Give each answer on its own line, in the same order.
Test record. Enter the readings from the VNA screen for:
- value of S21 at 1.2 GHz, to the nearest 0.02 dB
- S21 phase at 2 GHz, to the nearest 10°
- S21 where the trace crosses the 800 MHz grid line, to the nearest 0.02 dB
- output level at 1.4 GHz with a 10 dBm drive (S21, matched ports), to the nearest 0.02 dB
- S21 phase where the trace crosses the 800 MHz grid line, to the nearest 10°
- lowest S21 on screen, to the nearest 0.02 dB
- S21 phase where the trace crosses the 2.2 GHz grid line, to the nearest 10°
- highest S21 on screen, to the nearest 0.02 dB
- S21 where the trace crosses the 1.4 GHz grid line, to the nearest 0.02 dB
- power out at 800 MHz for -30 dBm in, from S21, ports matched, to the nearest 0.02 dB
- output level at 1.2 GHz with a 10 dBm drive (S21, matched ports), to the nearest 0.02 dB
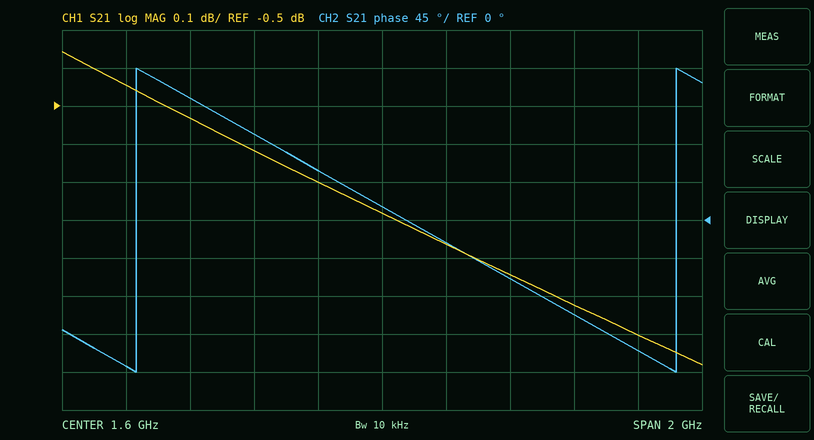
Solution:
-0.62 dB
-70°
-0.44 dB
9.30 dBm
-170°
-1.18 dB
-110°
-0.36 dB
-0.70 dB
-30.44 dBm
9.38 dBm
